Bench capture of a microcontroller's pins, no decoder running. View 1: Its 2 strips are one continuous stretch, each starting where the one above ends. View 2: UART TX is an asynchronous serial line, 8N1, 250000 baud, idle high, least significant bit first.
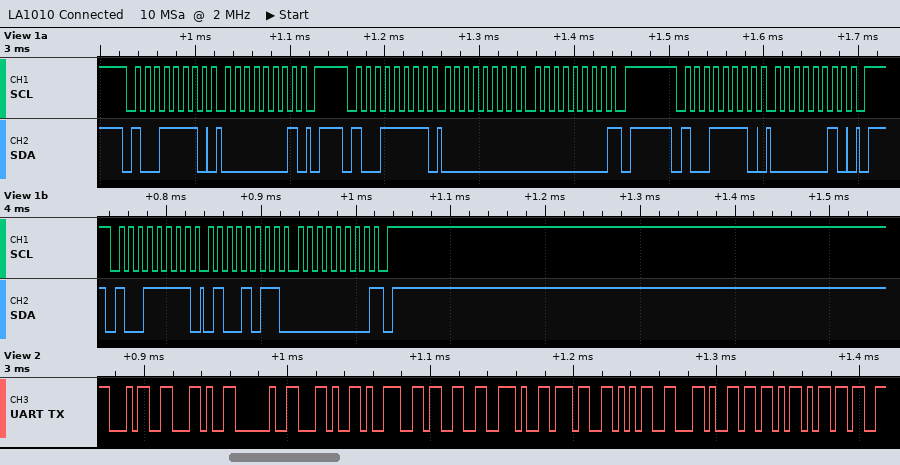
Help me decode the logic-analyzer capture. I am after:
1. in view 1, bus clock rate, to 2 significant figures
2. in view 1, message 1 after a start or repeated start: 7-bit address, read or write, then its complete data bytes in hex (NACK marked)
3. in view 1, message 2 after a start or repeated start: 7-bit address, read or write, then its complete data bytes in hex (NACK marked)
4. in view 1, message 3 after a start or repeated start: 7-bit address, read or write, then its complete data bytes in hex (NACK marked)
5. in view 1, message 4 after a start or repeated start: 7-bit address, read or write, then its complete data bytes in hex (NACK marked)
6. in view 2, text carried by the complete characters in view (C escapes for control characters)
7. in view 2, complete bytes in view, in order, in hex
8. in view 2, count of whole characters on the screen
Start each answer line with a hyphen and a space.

- 100 kHz
- 0x4F write: 01
- 0x4F read: 00 00 NACK
- 0x4F write: 02
- 0x4F read: 4B 00 NACK
- "4, ,93.75,[m"
- 34 2C 20 2C 39 33 2E 37 35 2C 5B 6D
- 12
